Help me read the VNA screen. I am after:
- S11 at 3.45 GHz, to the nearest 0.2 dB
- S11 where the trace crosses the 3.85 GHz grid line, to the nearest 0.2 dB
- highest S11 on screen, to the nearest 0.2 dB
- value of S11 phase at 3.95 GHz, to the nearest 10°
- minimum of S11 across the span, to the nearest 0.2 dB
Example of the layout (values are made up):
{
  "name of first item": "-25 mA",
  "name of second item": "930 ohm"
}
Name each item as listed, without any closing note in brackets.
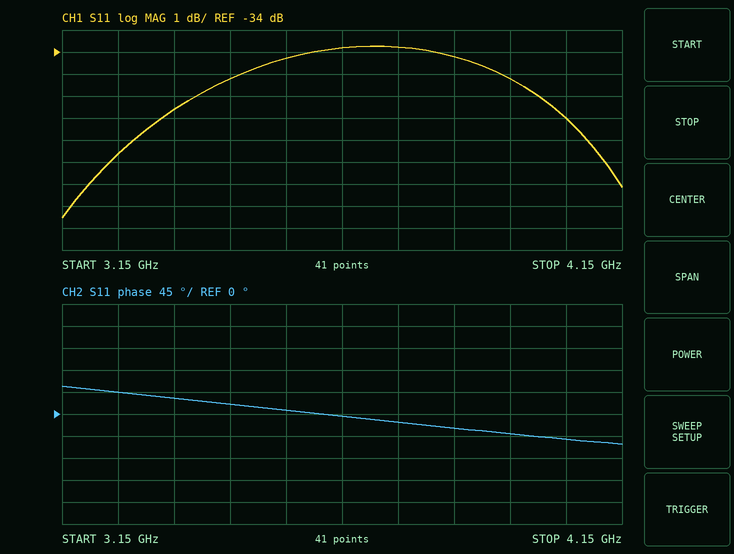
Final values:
{
  "S11 at 3.45 GHz, to the nearest 0.2 dB": "-35.2 dB",
  "S11 where the trace crosses the 3.85 GHz grid line, to the nearest 0.2 dB": "-34.2 dB",
  "highest S11 on screen, to the nearest 0.2 dB": "-33.8 dB",
  "value of S11 phase at 3.95 GHz, to the nearest 10°": "-40°",
  "minimum of S11 across the span, to the nearest 0.2 dB": "-41.6 dB"
}
